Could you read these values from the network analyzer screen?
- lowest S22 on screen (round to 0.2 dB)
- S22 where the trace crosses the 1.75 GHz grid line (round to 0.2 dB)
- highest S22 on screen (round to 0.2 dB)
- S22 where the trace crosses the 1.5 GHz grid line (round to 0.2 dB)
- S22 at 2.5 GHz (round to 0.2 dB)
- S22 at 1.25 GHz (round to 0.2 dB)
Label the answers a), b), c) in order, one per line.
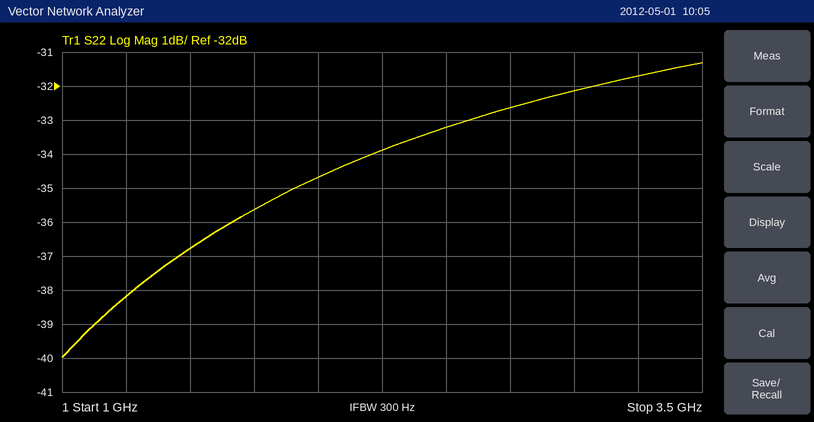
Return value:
a) -40.0 dB
b) -35.6 dB
c) -31.4 dB
d) -36.8 dB
e) -33.2 dB
f) -38.2 dB
